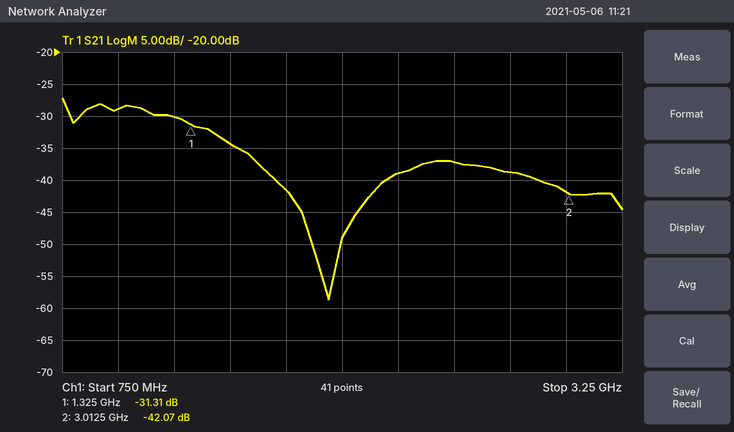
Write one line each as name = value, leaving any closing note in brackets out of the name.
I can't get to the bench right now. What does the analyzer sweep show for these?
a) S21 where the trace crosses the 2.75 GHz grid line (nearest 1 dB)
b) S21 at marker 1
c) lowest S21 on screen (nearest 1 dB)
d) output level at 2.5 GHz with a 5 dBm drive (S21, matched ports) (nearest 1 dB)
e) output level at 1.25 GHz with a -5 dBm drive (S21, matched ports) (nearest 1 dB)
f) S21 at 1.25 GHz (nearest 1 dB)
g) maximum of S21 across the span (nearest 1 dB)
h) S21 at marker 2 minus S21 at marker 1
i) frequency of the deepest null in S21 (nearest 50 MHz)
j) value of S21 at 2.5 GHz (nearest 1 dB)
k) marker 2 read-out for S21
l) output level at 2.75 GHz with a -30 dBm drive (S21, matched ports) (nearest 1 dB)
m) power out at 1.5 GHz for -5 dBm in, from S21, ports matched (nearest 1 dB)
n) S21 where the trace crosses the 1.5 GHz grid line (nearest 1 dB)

S21 where the trace crosses the 2.75 GHz grid line = -39 dB
S21 at marker 1 = -31.31 dB
lowest S21 on screen = -59 dB
output level at 2.5 GHz with a 5 dBm drive (S21, matched ports) = -32 dBm
output level at 1.25 GHz with a -5 dBm drive (S21, matched ports) = -35 dBm
S21 at 1.25 GHz = -30 dB
maximum of S21 across the span = -27 dB
S21 at marker 2 minus S21 at marker 1 = -10.76 dB
frequency of the deepest null in S21 = 1.95 GHz
value of S21 at 2.5 GHz = -37 dB
marker 2 read-out for S21 = -42.07 dB
output level at 2.75 GHz with a -30 dBm drive (S21, matched ports) = -69 dBm
power out at 1.5 GHz for -5 dBm in, from S21, ports matched = -39 dBm
S21 where the trace crosses the 1.5 GHz grid line = -34 dB
